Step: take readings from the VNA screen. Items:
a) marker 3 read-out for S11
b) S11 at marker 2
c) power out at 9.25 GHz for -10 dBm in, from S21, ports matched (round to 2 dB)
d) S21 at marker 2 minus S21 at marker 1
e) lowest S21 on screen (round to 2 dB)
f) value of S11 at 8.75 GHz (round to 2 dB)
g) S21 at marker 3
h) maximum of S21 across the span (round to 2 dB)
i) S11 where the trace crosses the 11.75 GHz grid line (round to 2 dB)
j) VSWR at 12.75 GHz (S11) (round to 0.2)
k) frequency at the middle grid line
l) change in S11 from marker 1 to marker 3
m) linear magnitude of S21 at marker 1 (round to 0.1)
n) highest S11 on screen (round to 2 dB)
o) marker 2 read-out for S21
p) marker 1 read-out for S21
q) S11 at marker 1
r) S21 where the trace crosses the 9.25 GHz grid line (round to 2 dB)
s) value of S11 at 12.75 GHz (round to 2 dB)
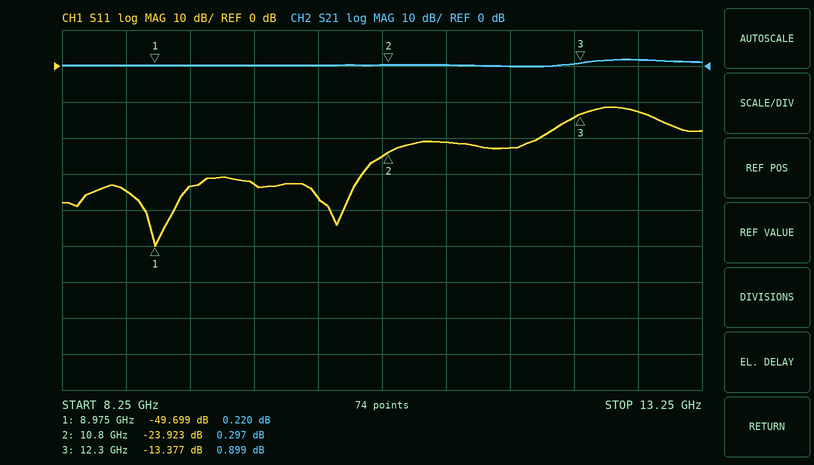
-13.377 dB
-23.923 dB
-10 dBm
0.077 dB
0 dB
-34 dB
0.899 dB
2 dB
-22 dB
1.6
10.75 GHz
36.322 dB
1.0
-12 dB
0.297 dB
0.220 dB
-49.699 dB
0 dB
-12 dB
